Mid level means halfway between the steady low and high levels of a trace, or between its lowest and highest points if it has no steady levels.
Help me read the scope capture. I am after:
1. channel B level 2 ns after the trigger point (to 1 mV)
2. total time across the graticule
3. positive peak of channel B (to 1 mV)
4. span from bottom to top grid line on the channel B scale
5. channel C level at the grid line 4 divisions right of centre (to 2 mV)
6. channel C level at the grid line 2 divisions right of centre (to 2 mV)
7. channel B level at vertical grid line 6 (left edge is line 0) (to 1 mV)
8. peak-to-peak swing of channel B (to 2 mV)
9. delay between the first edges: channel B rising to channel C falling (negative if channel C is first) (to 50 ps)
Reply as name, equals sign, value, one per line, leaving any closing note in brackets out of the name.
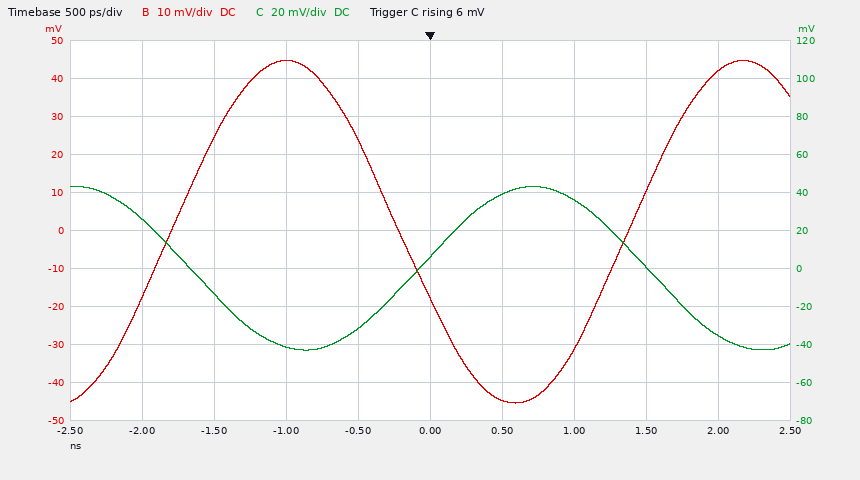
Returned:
channel B level 2 ns after the trigger point = 42 mV
total time across the graticule = 5 ns
positive peak of channel B = 45 mV
span from bottom to top grid line on the channel B scale = 100 mV
channel C level at the grid line 4 divisions right of centre = -36 mV
channel C level at the grid line 2 divisions right of centre = 36 mV
channel B level at vertical grid line 6 (left edge is line 0) = -45 mV
peak-to-peak swing of channel B = 90 mV
delay between the first edges: channel B rising to channel C falling (negative if channel C is first) = +150 ps
